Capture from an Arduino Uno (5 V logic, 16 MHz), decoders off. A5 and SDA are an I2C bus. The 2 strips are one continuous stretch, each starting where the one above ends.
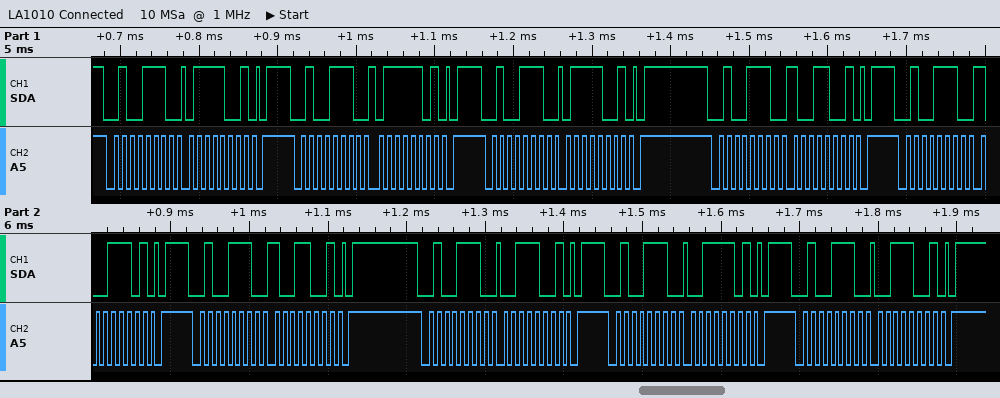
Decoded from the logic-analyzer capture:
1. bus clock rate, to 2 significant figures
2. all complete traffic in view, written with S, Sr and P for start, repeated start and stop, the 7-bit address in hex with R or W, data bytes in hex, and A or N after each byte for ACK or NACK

100 kHz
S 27W A 79 A P S 27W A 7D A P S 27W A 79 A P S 27W A 99 A P S 27W A 9D A P S 27W A 99 A P S 27W A 39 A P S 27W A 3D A P S 27W A 39 A P
